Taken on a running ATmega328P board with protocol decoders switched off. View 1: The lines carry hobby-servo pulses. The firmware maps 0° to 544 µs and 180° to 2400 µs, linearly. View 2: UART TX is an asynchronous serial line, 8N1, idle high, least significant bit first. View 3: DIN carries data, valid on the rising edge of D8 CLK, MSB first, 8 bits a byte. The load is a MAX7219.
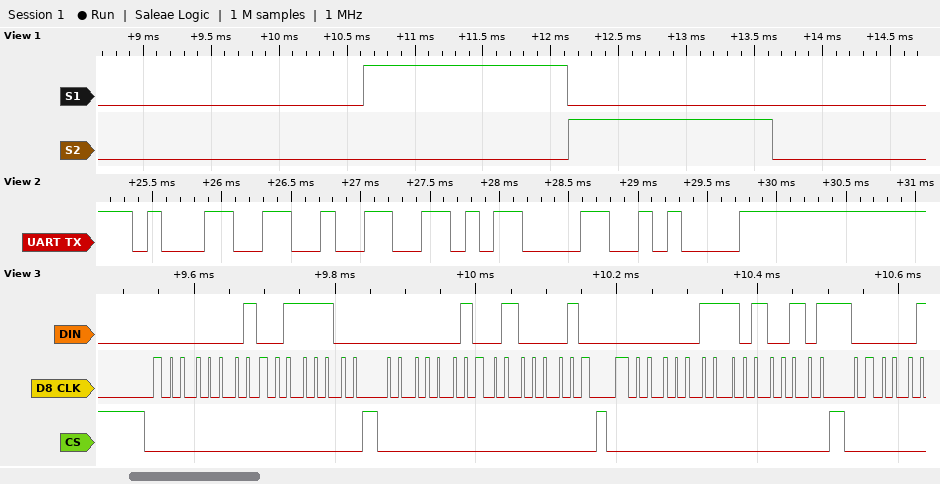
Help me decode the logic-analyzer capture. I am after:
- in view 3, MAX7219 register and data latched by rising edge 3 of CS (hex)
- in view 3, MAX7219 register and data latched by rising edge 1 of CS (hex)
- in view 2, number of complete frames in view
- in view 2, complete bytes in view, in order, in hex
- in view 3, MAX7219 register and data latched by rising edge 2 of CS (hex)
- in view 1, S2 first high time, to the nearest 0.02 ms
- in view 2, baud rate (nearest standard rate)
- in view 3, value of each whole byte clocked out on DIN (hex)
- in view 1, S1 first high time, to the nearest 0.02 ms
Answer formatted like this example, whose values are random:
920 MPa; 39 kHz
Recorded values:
register 0x3, data 0xA5; register 0x1, data 0x3C; 4; 31 32 0D 0A; register 0x2, data 0x42; 1.50 ms; 9600 baud; 01 3C 02 42 03 A5; 1.50 ms
